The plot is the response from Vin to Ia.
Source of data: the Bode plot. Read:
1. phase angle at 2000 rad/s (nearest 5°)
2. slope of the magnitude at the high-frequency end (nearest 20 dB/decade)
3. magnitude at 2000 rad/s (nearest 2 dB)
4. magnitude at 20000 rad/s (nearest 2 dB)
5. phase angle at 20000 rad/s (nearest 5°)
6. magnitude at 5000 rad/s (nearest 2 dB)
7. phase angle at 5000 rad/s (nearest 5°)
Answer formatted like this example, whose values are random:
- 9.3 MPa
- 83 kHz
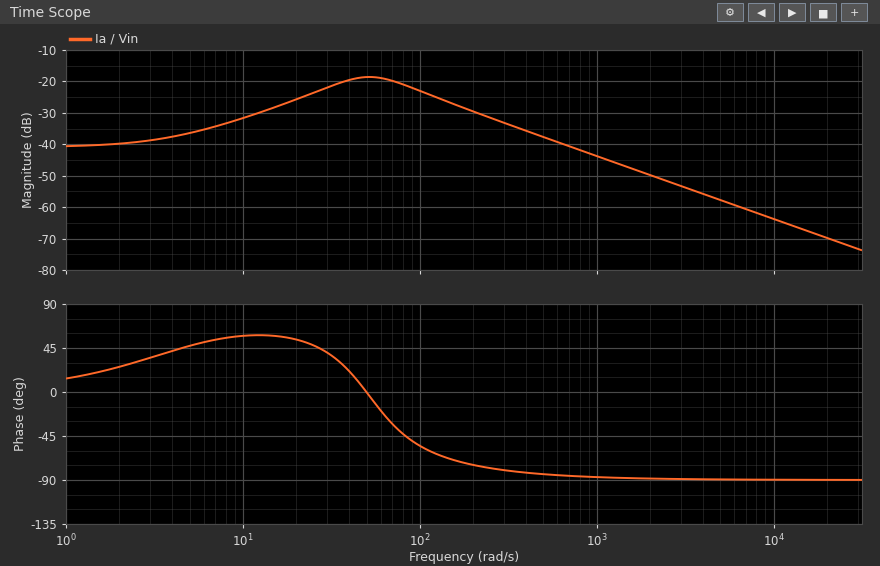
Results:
- -90°
- -20 dB/decade
- -50 dB
- -70 dB
- -90°
- -58 dB
- -90°
